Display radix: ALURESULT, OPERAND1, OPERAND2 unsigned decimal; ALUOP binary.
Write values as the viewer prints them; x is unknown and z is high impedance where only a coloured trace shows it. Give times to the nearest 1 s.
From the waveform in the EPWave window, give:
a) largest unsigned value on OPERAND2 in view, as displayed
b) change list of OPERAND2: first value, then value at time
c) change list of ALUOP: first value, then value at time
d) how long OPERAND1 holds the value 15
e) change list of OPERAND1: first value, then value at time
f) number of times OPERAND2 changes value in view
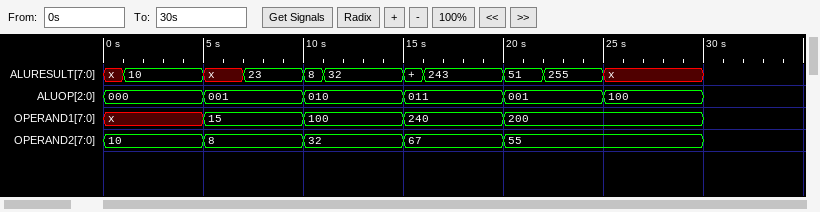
67
10, 8 at 5 s, 32 at 10 s, 67 at 15 s, 55 at 20 s
000, 001 at 5 s, 010 at 10 s, 011 at 15 s, 001 at 20 s, 100 at 25 s
5 s
x, 15 at 5 s, 100 at 10 s, 240 at 15 s, 200 at 20 s
4
